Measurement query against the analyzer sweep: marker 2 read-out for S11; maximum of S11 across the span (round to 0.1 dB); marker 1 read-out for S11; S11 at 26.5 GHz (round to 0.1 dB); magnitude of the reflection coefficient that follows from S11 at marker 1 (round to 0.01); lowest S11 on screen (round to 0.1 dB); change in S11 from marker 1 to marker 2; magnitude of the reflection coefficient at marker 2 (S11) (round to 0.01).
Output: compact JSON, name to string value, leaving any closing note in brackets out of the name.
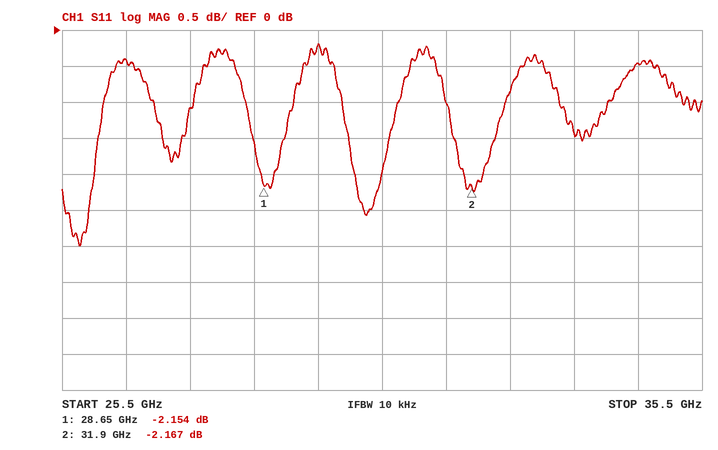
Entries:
{"marker 2 read-out for S11": "-2.167 dB", "maximum of S11 across the span": "-0.2 dB", "marker 1 read-out for S11": "-2.154 dB", "S11 at 26.5 GHz": "-0.4 dB", "magnitude of the reflection coefficient that follows from S11 at marker 1": "0.78", "lowest S11 on screen": "-3.0 dB", "change in S11 from marker 1 to marker 2": "-0.013 dB", "magnitude of the reflection coefficient at marker 2 (S11)": "0.78"}
